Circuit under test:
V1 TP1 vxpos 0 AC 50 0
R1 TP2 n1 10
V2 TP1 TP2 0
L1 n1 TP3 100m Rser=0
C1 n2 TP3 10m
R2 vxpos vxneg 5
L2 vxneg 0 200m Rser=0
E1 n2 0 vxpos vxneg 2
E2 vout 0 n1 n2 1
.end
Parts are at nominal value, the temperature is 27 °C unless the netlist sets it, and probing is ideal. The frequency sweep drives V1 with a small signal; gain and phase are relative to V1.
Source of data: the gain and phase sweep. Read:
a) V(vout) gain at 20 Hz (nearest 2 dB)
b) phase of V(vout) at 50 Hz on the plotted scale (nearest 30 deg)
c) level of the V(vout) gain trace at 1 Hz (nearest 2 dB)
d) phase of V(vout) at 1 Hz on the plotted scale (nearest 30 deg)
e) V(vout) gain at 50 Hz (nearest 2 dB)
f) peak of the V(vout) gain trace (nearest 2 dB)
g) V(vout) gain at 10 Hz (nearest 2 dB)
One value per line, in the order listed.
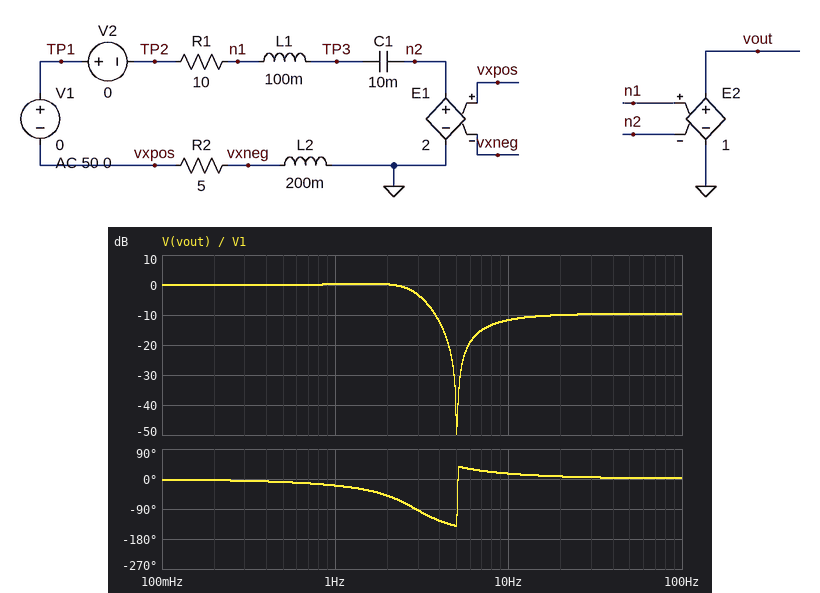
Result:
-10 dB
0 deg
0 dB
-30 deg
-10 dB
0 dB
-12 dB
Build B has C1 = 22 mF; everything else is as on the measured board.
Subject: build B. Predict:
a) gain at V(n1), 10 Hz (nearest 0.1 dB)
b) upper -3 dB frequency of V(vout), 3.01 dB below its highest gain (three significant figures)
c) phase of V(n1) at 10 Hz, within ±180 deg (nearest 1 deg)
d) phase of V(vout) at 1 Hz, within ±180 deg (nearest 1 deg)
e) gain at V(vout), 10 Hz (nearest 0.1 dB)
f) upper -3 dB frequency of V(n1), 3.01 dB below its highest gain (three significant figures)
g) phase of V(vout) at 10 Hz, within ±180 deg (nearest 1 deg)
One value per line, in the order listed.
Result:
-4.3 dB
1.53 Hz
76 deg
-43 deg
-10.6 dB
3.56 Hz
15 deg
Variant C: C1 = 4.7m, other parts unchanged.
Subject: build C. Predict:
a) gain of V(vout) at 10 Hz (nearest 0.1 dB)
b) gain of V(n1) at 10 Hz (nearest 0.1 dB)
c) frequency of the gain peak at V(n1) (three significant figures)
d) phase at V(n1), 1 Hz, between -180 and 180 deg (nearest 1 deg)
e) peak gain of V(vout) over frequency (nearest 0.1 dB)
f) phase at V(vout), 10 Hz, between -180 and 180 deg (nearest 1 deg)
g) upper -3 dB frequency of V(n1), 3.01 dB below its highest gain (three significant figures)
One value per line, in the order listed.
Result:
-15.0 dB
-3.9 dB
4.04 Hz
-26 deg
2.1 dB
18 deg
5.44 Hz
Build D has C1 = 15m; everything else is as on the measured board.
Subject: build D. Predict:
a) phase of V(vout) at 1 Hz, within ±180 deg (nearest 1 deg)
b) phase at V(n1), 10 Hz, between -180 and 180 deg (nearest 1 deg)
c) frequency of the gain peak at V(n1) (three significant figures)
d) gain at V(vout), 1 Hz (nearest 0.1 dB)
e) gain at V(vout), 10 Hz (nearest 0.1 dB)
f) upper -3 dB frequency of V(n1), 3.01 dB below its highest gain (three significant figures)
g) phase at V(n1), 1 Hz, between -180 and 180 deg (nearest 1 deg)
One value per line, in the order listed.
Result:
-30 deg
78 deg
2.24 Hz
-0.1 dB
-11.0 dB
3.86 Hz
-75 deg
